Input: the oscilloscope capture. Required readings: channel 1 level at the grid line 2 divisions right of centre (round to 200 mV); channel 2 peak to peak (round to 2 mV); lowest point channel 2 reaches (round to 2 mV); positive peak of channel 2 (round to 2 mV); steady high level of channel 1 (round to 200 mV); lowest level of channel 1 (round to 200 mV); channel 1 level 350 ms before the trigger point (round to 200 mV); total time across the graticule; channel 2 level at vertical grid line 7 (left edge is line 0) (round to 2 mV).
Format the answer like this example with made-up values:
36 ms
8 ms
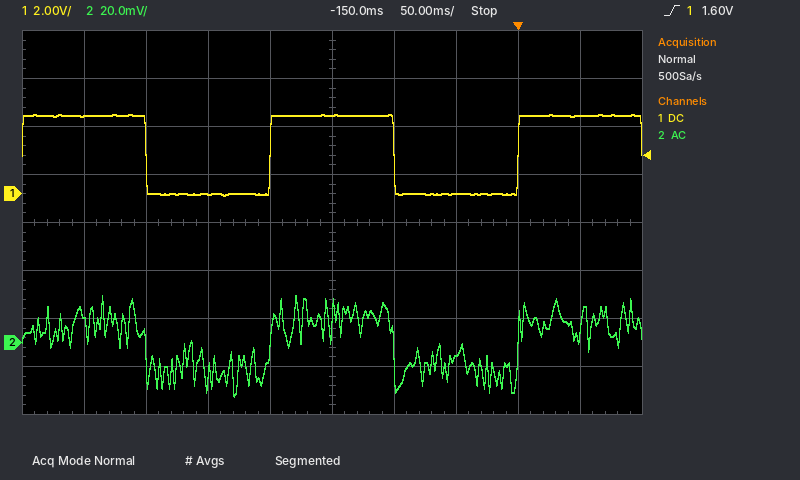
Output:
0.0 V
42 mV
-22 mV
20 mV
3.2 V
0.0 V
3.2 V
500 ms
-6 mV
